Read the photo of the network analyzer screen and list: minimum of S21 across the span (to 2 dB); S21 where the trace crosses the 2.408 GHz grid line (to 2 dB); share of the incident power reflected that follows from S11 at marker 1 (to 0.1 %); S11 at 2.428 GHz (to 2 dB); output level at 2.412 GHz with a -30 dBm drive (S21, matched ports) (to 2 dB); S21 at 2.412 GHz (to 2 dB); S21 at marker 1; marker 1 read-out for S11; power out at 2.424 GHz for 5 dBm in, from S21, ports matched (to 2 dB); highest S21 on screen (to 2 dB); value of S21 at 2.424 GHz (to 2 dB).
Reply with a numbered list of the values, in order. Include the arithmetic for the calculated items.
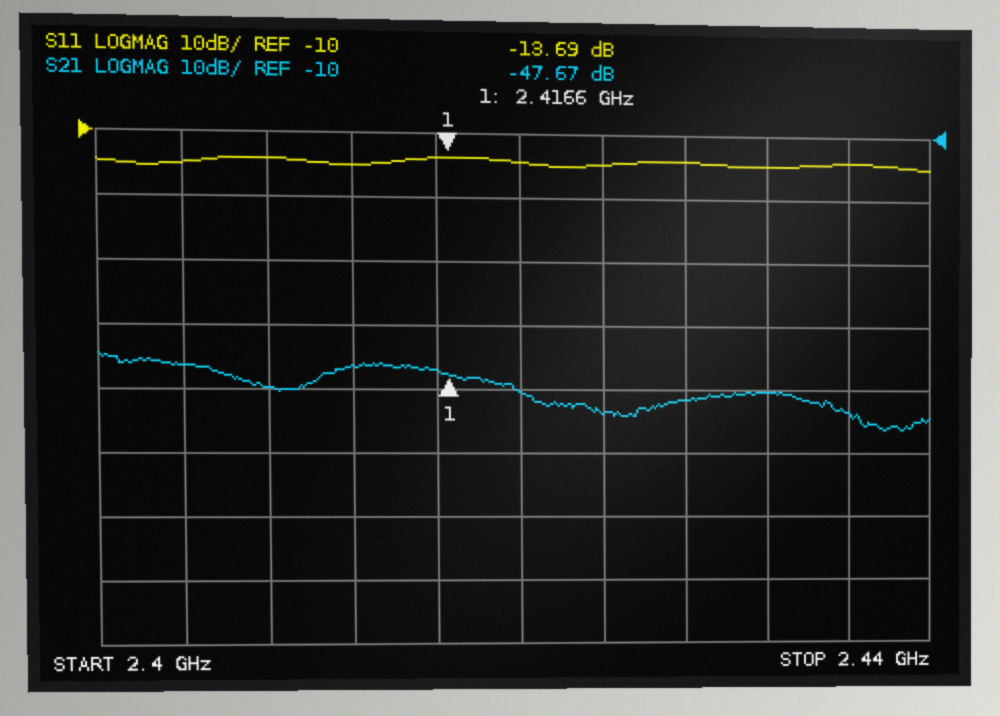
1. -56 dB
2. -50 dB
3. 10^(-13.69/10) ≈ 4.3 %
4. -14 dB
5. -30 dBm + (-46 dB) = -76 dBm
6. -46 dB
7. -47.67 dB
8. -13.69 dB
9. 5 dBm + (-54 dB) = -48 dBm
10. -44 dB
11. -54 dB
